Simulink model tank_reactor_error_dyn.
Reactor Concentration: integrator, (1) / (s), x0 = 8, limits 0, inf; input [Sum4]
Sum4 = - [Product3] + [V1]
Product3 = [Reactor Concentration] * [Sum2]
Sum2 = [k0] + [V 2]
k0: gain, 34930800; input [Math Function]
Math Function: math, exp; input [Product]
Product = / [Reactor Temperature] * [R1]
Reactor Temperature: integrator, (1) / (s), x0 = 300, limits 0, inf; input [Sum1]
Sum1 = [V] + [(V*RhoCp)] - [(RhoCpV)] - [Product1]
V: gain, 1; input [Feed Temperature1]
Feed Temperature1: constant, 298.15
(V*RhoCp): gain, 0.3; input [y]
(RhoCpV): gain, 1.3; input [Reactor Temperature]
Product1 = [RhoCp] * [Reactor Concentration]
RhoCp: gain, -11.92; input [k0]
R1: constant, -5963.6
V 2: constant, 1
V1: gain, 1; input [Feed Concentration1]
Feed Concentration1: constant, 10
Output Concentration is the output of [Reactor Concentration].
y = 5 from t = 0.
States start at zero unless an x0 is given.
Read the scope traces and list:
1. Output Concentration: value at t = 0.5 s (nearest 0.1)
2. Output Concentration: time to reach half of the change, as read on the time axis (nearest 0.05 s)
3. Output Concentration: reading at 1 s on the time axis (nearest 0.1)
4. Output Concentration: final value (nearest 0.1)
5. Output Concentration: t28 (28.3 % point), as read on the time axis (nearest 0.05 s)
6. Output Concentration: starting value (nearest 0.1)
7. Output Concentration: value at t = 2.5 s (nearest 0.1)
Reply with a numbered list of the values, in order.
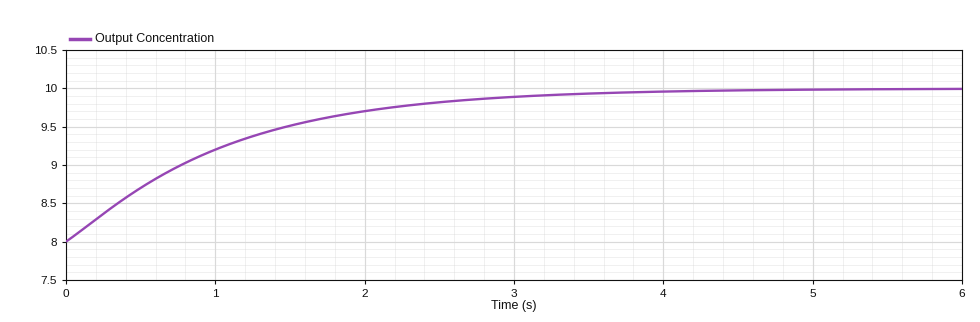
1. 8.7
2. 0.75 s
3. 9.2
4. 10.0
5. 0.40 s
6. 8.0
7. 9.8
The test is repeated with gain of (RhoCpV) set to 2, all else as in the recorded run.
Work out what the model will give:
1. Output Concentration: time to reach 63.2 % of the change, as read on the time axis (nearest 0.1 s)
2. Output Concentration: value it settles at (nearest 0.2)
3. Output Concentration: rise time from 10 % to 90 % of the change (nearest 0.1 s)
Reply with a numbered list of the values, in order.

1. 1.0 s
2. 10.0
3. 2.2 s
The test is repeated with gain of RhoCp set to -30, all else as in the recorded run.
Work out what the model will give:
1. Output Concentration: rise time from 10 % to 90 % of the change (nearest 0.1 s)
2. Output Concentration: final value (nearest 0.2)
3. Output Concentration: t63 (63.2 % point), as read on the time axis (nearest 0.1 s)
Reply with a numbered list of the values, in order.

1. 2.3 s
2. 10.0
3. 1.1 s
